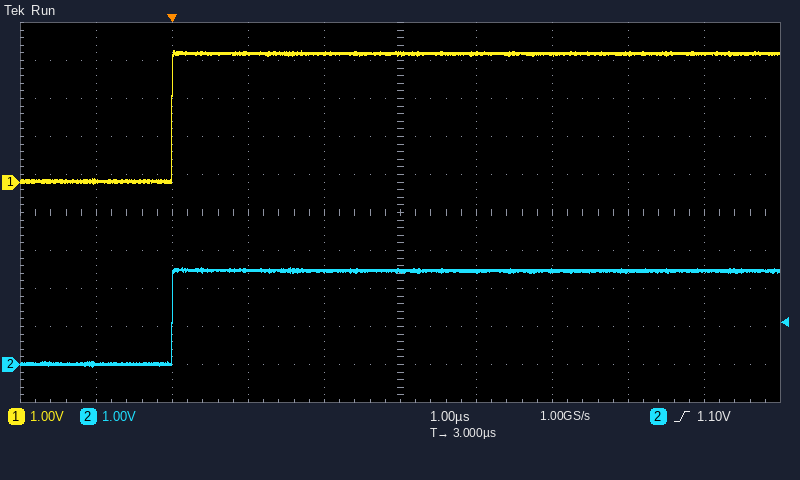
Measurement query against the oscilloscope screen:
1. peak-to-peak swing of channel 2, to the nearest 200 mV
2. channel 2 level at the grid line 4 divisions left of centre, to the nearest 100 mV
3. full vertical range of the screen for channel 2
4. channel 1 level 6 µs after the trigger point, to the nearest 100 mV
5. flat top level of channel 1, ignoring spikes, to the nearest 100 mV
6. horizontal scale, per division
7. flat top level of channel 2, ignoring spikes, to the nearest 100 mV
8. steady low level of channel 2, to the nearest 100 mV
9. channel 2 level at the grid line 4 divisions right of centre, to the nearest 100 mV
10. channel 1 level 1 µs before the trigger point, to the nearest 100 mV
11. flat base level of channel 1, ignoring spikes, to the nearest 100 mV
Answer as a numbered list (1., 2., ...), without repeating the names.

1. 2.6 V
2. 0.0 V
3. 10 V
4. 3.4 V
5. 3.4 V
6. 1 µs
7. 2.5 V
8. 0.0 V
9. 2.5 V
10. 0.0 V
11. 0.0 V
